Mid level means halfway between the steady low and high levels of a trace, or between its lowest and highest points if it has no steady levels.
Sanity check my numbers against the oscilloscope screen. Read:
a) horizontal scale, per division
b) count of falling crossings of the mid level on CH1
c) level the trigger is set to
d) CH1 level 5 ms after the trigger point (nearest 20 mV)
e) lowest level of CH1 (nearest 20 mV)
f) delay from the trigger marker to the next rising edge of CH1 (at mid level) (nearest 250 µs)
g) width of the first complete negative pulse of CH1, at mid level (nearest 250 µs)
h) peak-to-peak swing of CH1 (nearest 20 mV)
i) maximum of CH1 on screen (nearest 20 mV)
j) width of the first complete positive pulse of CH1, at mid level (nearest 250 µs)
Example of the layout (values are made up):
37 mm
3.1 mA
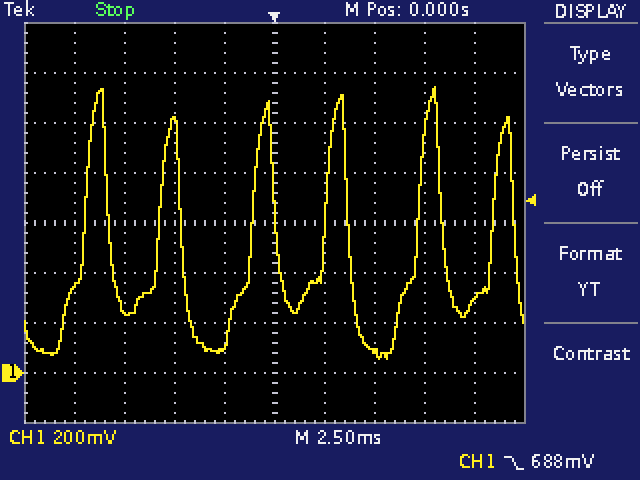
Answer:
2.5 ms
6
688 mV
80 mV
60 mV
2.50 ms
2.50 ms
1.08 V
1.14 V
1.25 ms
